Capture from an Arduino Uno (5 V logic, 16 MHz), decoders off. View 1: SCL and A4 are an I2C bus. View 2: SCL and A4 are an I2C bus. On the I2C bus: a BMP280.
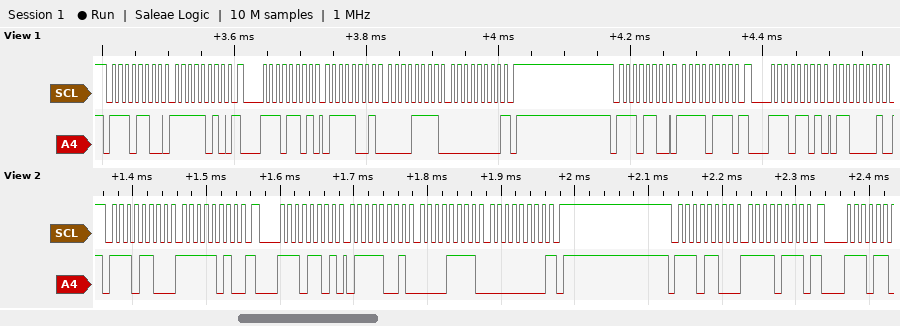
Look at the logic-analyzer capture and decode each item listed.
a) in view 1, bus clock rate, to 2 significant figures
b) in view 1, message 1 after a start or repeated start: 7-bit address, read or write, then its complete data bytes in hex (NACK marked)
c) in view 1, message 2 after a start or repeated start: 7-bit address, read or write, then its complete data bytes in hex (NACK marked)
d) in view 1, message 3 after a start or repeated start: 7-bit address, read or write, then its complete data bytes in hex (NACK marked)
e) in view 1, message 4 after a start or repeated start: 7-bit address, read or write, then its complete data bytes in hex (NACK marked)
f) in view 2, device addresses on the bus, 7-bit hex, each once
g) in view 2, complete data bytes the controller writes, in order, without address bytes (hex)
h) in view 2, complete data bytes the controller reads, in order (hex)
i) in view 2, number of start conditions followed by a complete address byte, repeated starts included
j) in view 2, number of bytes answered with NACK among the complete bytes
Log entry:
100 kHz
0x76 write: FA
0x76 read: 79 0F 00 NACK
0x76 write: F7
0x76 read: 61
0x76
FA F7
79 0F 00
3
1
